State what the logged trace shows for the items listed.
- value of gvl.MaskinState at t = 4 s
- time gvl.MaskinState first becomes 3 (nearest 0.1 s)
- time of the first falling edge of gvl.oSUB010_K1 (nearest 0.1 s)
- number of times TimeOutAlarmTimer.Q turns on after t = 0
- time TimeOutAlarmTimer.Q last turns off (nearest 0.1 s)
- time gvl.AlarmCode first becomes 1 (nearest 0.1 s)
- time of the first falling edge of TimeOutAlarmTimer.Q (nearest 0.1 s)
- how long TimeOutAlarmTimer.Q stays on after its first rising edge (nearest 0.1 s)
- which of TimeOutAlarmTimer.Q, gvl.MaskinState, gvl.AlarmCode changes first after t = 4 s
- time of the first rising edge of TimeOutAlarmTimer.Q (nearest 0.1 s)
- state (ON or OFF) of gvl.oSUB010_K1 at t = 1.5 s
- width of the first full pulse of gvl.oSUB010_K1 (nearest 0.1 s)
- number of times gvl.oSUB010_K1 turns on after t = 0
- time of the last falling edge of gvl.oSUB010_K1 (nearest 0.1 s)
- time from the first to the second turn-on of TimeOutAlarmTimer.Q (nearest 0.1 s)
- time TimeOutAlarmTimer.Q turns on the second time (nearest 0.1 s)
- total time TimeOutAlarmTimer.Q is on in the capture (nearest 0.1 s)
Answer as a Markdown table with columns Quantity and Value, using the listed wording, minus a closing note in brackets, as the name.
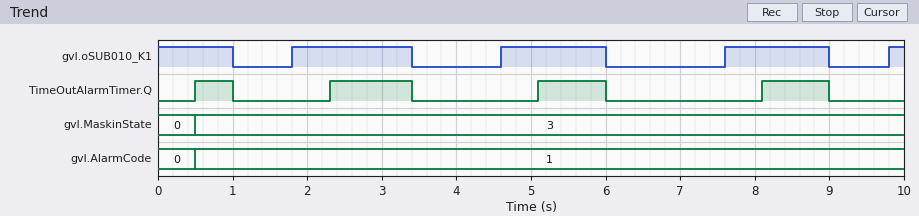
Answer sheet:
| Quantity | Value |
|---|---|
| value of gvl.MaskinState at t = 4 s | 3 |
| time gvl.MaskinState first becomes 3 | 0.5 s |
| time of the first falling edge of gvl.oSUB010_K1 | 1.0 s |
| number of times TimeOutAlarmTimer.Q turns on after t = 0 | 4 |
| time TimeOutAlarmTimer.Q last turns off | 9.0 s |
| time gvl.AlarmCode first becomes 1 | 0.5 s |
| time of the first falling edge of TimeOutAlarmTimer.Q | 1.0 s |
| how long TimeOutAlarmTimer.Q stays on after its first rising edge | 0.5 s |
| which of TimeOutAlarmTimer.Q, gvl.MaskinState, gvl.AlarmCode changes first after t = 4 s | TimeOutAlarmTimer.Q |
| time of the first rising edge of TimeOutAlarmTimer.Q | 0.5 s |
| state (ON or OFF) of gvl.oSUB010_K1 at t = 1.5 s | OFF |
| width of the first full pulse of gvl.oSUB010_K1 | 1.6 s |
| number of times gvl.oSUB010_K1 turns on after t = 0 | 4 |
| time of the last falling edge of gvl.oSUB010_K1 | 9.0 s |
| time from the first to the second turn-on of TimeOutAlarmTimer.Q | 1.8 s |
| time TimeOutAlarmTimer.Q turns on the second time | 2.3 s |
| total time TimeOutAlarmTimer.Q is on in the capture | 3.4 s |
